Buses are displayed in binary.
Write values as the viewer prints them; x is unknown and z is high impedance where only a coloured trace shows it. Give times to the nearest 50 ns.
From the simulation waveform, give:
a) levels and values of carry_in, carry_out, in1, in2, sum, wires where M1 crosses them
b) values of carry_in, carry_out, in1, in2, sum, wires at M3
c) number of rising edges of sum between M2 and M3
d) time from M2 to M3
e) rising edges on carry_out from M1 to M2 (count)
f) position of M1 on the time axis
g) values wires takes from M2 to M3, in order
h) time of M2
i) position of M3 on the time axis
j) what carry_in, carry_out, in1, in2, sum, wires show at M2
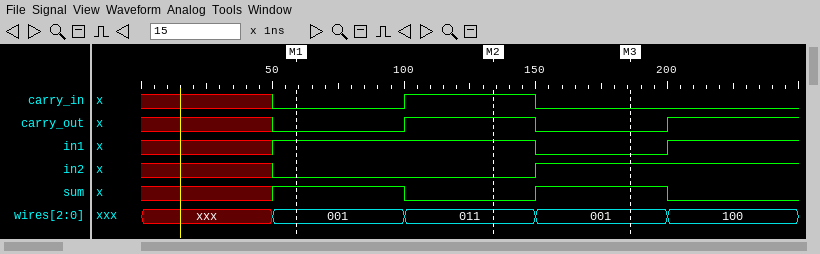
carry_in=0, carry_out=0, in1=1, in2=0, sum=1, wires=001
carry_in=0, carry_out=0, in1=0, in2=1, sum=1, wires=001
1
50 ns
1
50 ns
011, 001
150 ns
200 ns
carry_in=1, carry_out=1, in1=1, in2=0, sum=0, wires=011
